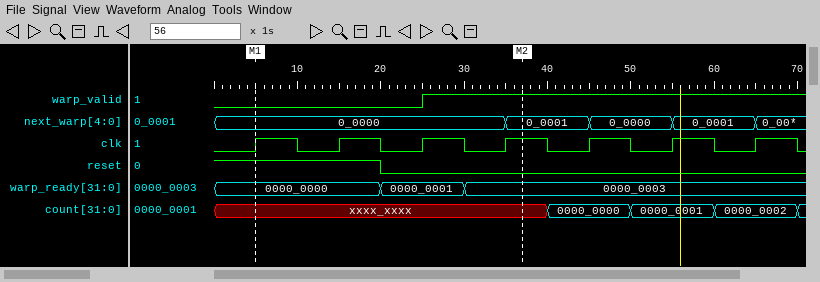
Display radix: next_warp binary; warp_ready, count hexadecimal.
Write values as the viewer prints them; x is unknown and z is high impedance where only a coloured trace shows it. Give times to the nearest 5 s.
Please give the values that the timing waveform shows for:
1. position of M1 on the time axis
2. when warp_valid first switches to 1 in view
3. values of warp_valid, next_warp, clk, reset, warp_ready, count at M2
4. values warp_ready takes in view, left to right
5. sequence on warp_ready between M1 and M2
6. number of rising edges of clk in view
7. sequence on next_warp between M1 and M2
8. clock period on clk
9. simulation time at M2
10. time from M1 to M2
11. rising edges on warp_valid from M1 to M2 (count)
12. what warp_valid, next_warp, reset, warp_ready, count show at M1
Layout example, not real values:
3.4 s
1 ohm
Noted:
5 s
25 s
warp_valid=1, next_warp=0_0001, clk=1, reset=0, warp_ready=0000_0003, count=xxxx_xxxx
0000_0000, 0000_0001, 0000_0003
0000_0000, 0000_0001, 0000_0003
7
0_0000, 0_0001
10 s
35 s
30 s
1
warp_valid=0, next_warp=0_0000, reset=1, warp_ready=0000_0000, count=xxxx_xxxx
